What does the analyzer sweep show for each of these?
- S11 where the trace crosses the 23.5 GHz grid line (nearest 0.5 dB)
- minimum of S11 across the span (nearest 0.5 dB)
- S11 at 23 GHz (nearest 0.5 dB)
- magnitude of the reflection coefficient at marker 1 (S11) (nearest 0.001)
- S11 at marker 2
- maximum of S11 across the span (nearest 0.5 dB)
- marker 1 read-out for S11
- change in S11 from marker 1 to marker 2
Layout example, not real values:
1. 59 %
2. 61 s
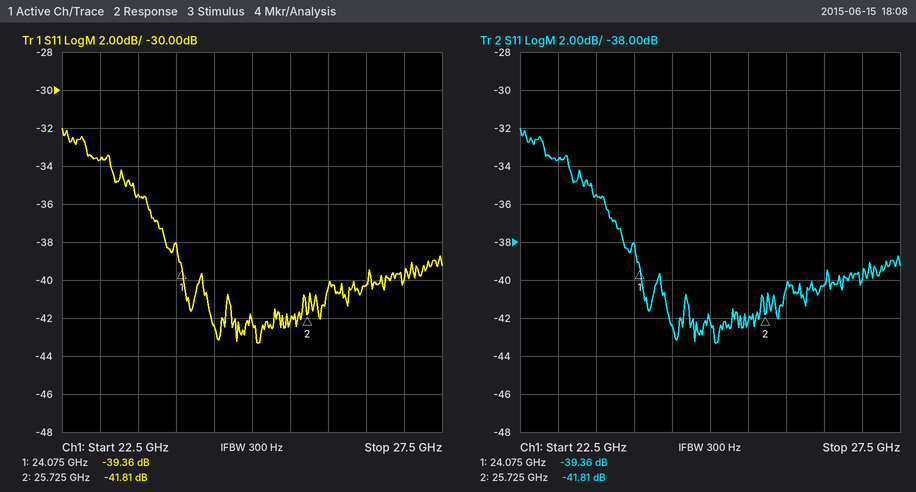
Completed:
1. -35.5 dB
2. -43.5 dB
3. -33.5 dB
4. 0.011
5. -41.81 dB
6. -32.0 dB
7. -39.36 dB
8. -2.45 dB
